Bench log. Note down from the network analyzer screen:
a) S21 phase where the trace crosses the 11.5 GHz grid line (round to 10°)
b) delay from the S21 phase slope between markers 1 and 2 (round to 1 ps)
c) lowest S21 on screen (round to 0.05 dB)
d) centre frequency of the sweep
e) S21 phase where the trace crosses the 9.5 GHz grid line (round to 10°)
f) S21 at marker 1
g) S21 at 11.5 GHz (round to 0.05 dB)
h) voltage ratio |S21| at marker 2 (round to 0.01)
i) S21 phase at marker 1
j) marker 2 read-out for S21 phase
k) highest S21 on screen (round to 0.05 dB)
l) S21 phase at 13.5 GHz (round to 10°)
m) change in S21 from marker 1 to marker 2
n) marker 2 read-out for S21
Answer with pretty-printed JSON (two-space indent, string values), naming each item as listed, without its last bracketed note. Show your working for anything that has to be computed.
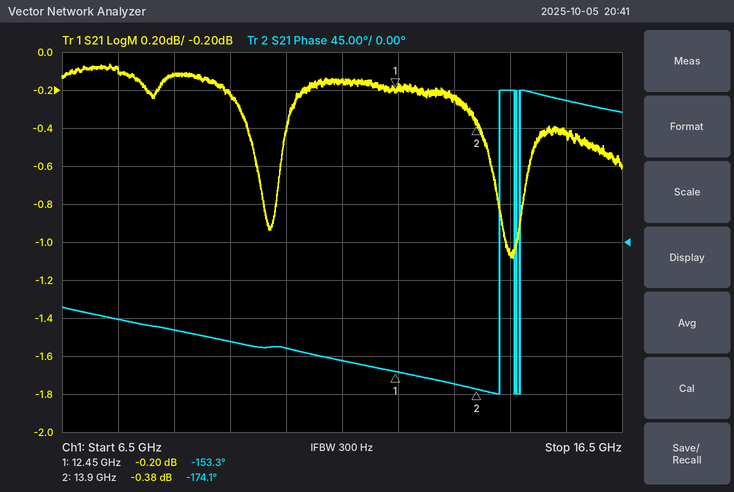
{
  "S21 phase where the trace crosses the 11.5 GHz grid line": "-140°",
  "delay from the S21 phase slope between markers 1 and 2": "−(-174.1° − (-153.3°))/(360° × 1.45 GHz) ≈ 40 ps",
  "lowest S21 on screen": "-1.10 dB",
  "centre frequency of the sweep": "11.5 GHz",
  "S21 phase where the trace crosses the 9.5 GHz grid line": "-120°",
  "S21 at marker 1": "-0.20 dB",
  "S21 at 11.5 GHz": "-0.15 dB",
  "voltage ratio |S21| at marker 2": "10^(-0.38/20) ≈ 0.96",
  "S21 phase at marker 1": "-153.3°",
  "marker 2 read-out for S21 phase": "-174.1°",
  "highest S21 on screen": "-0.05 dB",
  "S21 phase at 13.5 GHz": "-170°",
  "change in S21 from marker 1 to marker 2": "-0.38 − (-0.2) = -0.18 dB",
  "marker 2 read-out for S21": "-0.38 dB"
}
